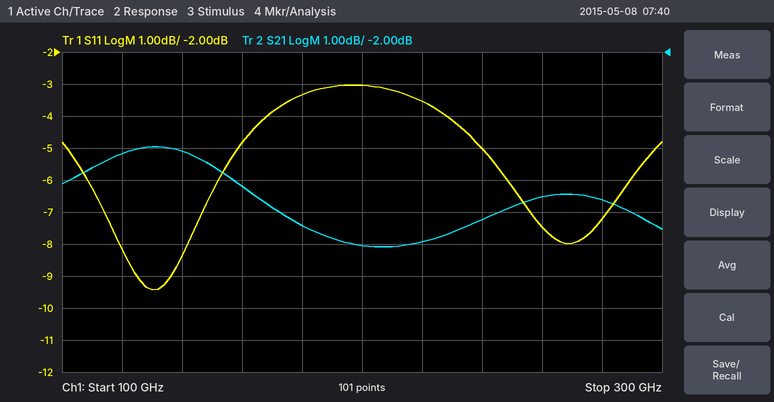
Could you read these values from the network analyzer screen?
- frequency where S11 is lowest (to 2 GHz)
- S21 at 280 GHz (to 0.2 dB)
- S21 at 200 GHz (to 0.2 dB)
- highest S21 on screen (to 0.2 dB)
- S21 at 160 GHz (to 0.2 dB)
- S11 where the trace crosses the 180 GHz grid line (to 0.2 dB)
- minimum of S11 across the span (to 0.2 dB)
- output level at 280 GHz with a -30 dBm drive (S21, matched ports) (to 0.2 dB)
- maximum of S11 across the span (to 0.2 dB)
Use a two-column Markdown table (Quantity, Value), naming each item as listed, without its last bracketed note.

| Quantity | Value |
|---|---|
| frequency where S11 is lowest | 130 GHz |
| S21 at 280 GHz | -6.6 dB |
| S21 at 200 GHz | -8.0 dB |
| highest S21 on screen | -5.0 dB |
| S21 at 160 GHz | -6.2 dB |
| S11 where the trace crosses the 180 GHz grid line | -3.4 dB |
| minimum of S11 across the span | -9.4 dB |
| output level at 280 GHz with a -30 dBm drive (S21, matched ports) | -36.6 dBm |
| maximum of S11 across the span | -3.0 dB |
